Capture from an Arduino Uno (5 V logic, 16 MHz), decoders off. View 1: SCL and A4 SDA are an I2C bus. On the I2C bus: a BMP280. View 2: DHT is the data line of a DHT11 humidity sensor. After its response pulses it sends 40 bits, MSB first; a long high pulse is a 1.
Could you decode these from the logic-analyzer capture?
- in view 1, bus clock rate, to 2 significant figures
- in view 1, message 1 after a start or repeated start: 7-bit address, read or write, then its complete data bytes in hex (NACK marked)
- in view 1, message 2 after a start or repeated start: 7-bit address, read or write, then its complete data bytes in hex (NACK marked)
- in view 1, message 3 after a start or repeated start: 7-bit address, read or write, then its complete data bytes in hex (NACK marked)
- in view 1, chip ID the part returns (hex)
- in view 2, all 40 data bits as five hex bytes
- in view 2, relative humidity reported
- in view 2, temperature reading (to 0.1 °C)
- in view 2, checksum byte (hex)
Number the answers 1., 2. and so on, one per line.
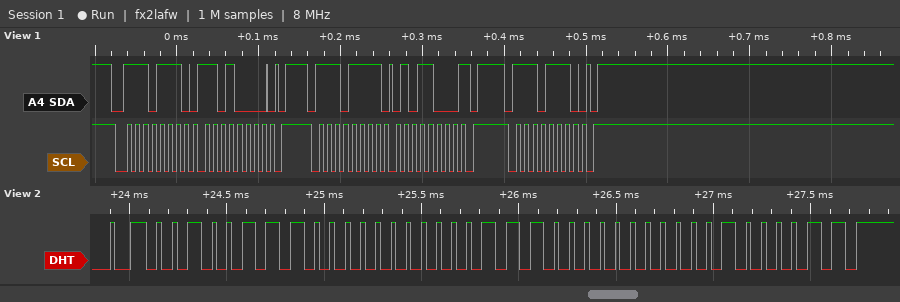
1. 100 kHz
2. 0x77 write: D0
3. 0x77 read: 58 NACK
4. 0x77 write
5. 0x58
6. 27 00 1C 00 43
7. 39 %
8. 28.0 °C
9. 0x43
